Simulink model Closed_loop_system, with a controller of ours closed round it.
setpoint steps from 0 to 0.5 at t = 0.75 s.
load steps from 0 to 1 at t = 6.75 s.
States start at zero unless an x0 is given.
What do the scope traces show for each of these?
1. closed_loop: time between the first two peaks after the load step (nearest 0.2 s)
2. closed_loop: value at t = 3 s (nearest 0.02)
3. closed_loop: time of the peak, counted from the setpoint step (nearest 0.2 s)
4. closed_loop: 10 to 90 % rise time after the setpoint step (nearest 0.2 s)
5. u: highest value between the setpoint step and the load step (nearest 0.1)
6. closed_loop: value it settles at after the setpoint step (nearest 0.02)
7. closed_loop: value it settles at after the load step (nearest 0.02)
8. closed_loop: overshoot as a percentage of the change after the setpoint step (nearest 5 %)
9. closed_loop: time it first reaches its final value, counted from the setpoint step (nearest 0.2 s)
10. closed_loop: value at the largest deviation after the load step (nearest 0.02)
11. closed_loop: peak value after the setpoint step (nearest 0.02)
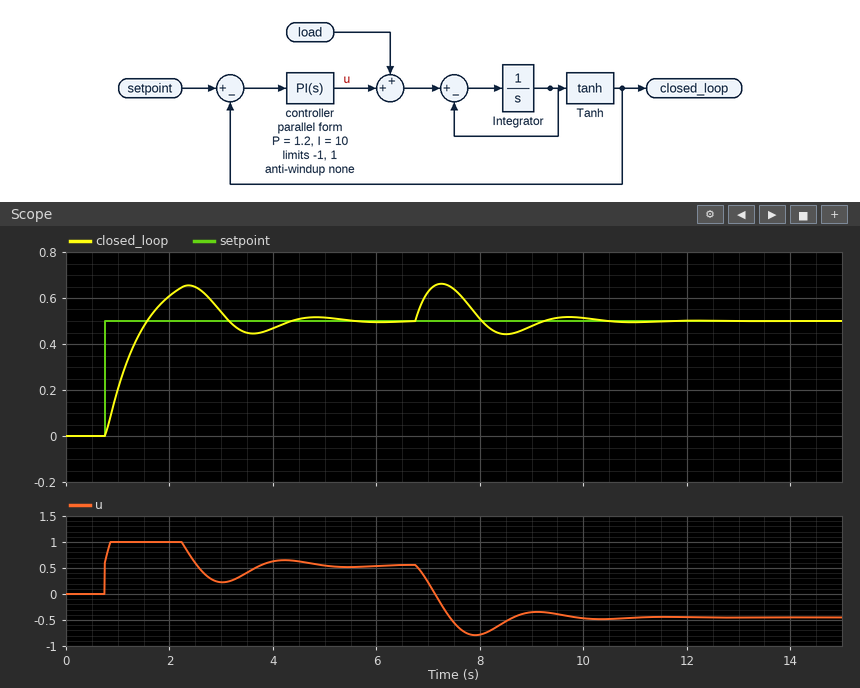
2.4 s
0.54
1.6 s
0.6 s
1.0
0.50
0.50
30 %
0.8 s
0.66
0.66
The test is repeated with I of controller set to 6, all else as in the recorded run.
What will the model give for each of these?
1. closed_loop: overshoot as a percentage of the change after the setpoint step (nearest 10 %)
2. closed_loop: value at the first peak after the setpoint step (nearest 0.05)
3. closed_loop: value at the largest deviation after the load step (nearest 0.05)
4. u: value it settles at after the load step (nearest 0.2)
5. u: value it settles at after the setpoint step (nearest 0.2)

20 %
0.60
0.70
-0.4
0.6
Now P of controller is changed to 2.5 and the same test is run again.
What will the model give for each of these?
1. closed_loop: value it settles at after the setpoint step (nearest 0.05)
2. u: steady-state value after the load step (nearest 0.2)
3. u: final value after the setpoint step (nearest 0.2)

0.50
-0.4
0.6
